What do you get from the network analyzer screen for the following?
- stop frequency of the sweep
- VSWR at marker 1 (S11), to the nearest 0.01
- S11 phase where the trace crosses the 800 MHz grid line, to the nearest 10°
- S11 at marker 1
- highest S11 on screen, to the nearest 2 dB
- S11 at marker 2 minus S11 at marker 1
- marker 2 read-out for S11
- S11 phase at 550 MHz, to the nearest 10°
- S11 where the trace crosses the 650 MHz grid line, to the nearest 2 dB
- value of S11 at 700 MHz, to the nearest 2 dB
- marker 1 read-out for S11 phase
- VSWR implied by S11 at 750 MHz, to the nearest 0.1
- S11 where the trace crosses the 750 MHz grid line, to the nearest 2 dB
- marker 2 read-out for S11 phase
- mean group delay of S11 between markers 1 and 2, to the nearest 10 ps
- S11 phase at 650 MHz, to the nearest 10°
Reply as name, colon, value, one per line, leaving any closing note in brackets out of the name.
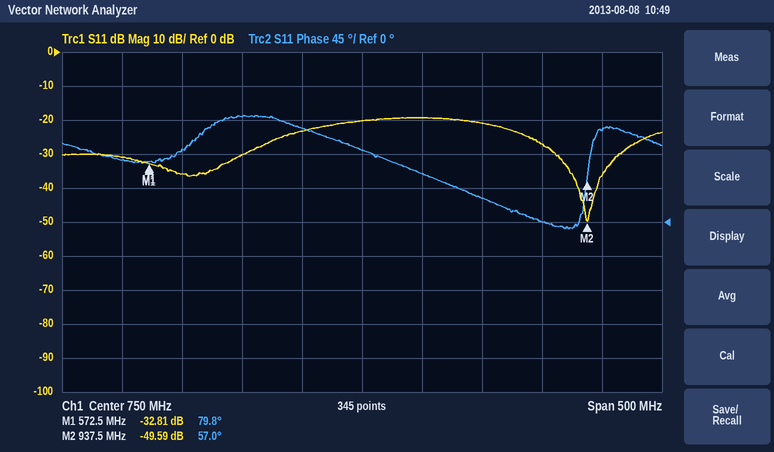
stop frequency of the sweep: 1 GHz
VSWR at marker 1 (S11), to the nearest 0.01: 1.05
S11 phase where the trace crosses the 800 MHz grid line, to the nearest 10°: 60°
S11 at marker 1: -32.81 dB
highest S11 on screen, to the nearest 2 dB: -20 dB
S11 at marker 2 minus S11 at marker 1: -16.78 dB
marker 2 read-out for S11: -49.59 dB
S11 phase at 550 MHz, to the nearest 10°: 80°
S11 where the trace crosses the 650 MHz grid line, to the nearest 2 dB: -30 dB
value of S11 at 700 MHz, to the nearest 2 dB: -24 dB
marker 1 read-out for S11 phase: 79.8°
VSWR implied by S11 at 750 MHz, to the nearest 0.1: 1.2
S11 where the trace crosses the 750 MHz grid line, to the nearest 2 dB: -20 dB
marker 2 read-out for S11 phase: 57.0°
mean group delay of S11 between markers 1 and 2, to the nearest 10 ps: 170 ps
S11 phase at 650 MHz, to the nearest 10°: 140°
